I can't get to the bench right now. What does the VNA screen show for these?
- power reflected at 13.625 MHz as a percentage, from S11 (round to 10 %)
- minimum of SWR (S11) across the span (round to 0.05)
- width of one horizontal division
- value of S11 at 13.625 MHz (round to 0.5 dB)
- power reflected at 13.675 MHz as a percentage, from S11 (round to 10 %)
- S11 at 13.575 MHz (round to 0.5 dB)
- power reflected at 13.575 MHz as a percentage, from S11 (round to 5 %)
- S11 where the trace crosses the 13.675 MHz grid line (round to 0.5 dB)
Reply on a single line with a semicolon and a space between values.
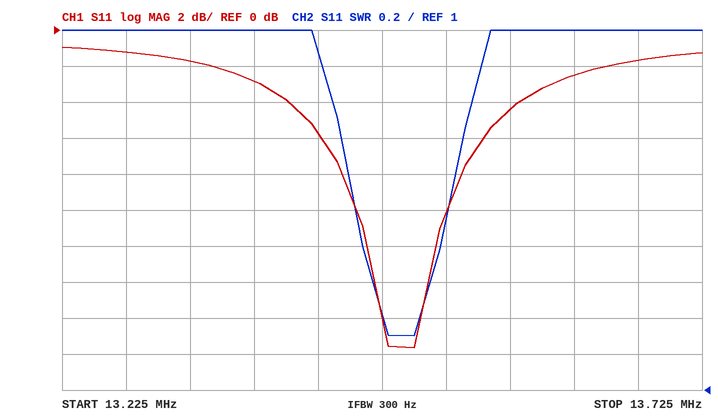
60 %; 1.30; 50 kHz; -2.5 dB; 70 %; -4.5 dB; 35 %; -1.5 dB
